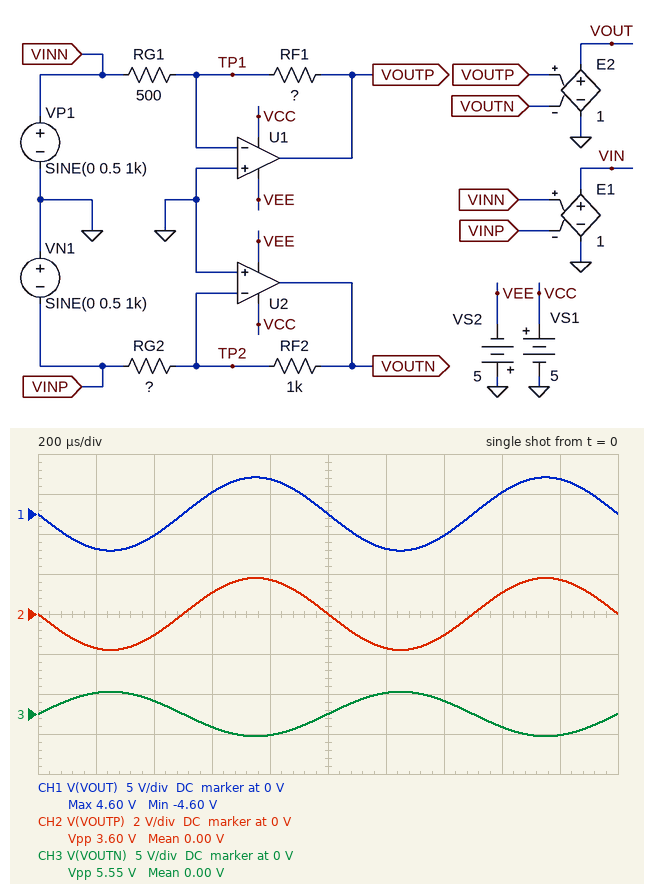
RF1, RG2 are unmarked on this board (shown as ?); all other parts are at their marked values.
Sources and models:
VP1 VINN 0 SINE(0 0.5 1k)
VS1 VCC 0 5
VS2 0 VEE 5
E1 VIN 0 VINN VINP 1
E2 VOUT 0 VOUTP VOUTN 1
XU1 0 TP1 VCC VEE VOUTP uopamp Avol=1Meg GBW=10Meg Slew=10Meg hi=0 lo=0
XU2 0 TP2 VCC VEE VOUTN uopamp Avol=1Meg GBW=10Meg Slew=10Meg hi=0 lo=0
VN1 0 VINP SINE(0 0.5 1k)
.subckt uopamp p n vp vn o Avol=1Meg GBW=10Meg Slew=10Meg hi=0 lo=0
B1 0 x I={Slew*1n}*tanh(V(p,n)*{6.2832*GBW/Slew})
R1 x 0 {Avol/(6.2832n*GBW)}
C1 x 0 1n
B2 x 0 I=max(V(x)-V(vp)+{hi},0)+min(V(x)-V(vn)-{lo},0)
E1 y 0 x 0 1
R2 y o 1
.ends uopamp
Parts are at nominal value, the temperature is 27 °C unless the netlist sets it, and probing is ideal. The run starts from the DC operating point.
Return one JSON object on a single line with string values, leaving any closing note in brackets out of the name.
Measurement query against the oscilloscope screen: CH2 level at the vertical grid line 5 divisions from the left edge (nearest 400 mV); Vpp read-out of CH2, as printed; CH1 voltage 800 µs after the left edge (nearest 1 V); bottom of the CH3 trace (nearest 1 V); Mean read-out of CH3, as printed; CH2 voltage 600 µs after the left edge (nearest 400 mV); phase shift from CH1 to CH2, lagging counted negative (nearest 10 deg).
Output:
{"CH2 level at the vertical grid line 5 divisions from the left edge": "0 V", "Vpp read-out of CH2, as printed": "3.60 V", "CH1 voltage 800 µs after the left edge": "4 V", "bottom of the CH3 trace": "-3 V", "Mean read-out of CH3, as printed": "0.00 V", "CH2 voltage 600 µs after the left edge": "1.2 V", "phase shift from CH1 to CH2, lagging counted negative": "0 deg"}
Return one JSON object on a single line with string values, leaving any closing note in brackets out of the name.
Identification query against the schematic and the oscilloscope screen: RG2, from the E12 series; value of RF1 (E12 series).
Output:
{"RG2, from the E12 series": "180 Ω", "value of RF1": "1.8 kΩ"}
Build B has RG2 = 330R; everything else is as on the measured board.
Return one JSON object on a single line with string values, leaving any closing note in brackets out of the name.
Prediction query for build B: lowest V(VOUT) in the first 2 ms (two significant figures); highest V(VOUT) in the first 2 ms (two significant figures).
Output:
{"lowest V(VOUT) in the first 2 ms": "-3.3 V", "highest V(VOUT) in the first 2 ms": "3.3 V"}
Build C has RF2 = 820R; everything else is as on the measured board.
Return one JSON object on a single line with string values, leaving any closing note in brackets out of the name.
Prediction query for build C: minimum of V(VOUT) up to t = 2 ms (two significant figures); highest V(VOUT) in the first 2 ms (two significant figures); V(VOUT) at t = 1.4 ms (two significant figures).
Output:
{"minimum of V(VOUT) up to t = 2 ms": "-4.1 V", "highest V(VOUT) in the first 2 ms": "4.1 V", "V(VOUT) at t = 1.4 ms": "-2.4 V"}
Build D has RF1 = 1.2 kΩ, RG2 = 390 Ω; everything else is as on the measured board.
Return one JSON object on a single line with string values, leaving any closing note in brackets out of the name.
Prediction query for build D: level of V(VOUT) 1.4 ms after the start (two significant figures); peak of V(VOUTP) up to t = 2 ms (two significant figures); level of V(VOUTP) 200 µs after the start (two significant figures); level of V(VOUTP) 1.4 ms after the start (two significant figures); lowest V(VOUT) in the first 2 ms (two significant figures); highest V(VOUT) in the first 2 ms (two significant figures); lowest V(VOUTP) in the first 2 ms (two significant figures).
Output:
{"level of V(VOUT) 1.4 ms after the start": "-1.5 V", "peak of V(VOUTP) up to t = 2 ms": "1.2 V", "level of V(VOUTP) 200 µs after the start": "-1.1 V", "level of V(VOUTP) 1.4 ms after the start": "-710 mV", "lowest V(VOUT) in the first 2 ms": "-2.5 V", "highest V(VOUT) in the first 2 ms": "2.5 V", "lowest V(VOUTP) in the first 2 ms": "-1.2 V"}
